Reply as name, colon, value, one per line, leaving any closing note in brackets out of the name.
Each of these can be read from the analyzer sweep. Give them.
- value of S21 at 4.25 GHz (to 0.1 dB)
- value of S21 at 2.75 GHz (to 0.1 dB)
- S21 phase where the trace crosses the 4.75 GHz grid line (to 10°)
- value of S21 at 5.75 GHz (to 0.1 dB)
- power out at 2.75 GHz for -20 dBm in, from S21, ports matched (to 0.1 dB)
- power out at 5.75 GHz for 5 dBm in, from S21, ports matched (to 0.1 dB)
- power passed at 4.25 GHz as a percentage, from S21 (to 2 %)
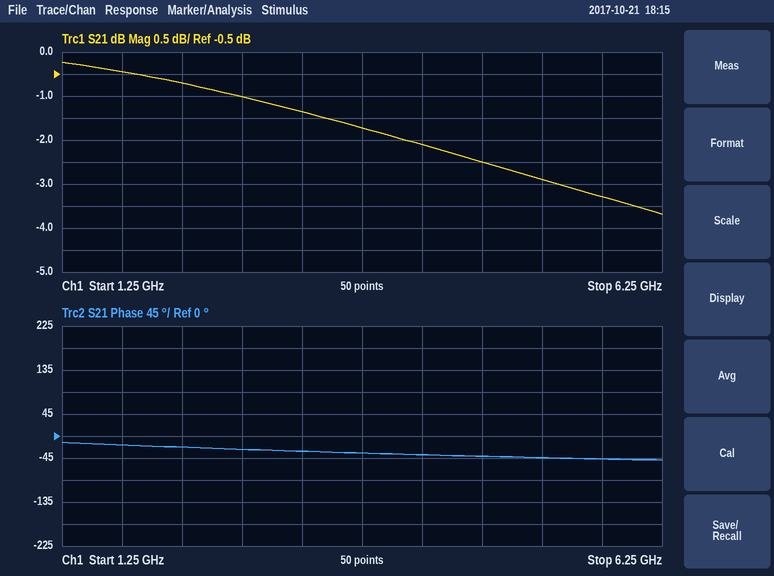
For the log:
value of S21 at 4.25 GHz: -2.1 dB
value of S21 at 2.75 GHz: -1.0 dB
S21 phase where the trace crosses the 4.75 GHz grid line: -40°
value of S21 at 5.75 GHz: -3.3 dB
power out at 2.75 GHz for -20 dBm in, from S21, ports matched: -21.0 dBm
power out at 5.75 GHz for 5 dBm in, from S21, ports matched: 1.7 dBm
power passed at 4.25 GHz as a percentage, from S21: 62 %
